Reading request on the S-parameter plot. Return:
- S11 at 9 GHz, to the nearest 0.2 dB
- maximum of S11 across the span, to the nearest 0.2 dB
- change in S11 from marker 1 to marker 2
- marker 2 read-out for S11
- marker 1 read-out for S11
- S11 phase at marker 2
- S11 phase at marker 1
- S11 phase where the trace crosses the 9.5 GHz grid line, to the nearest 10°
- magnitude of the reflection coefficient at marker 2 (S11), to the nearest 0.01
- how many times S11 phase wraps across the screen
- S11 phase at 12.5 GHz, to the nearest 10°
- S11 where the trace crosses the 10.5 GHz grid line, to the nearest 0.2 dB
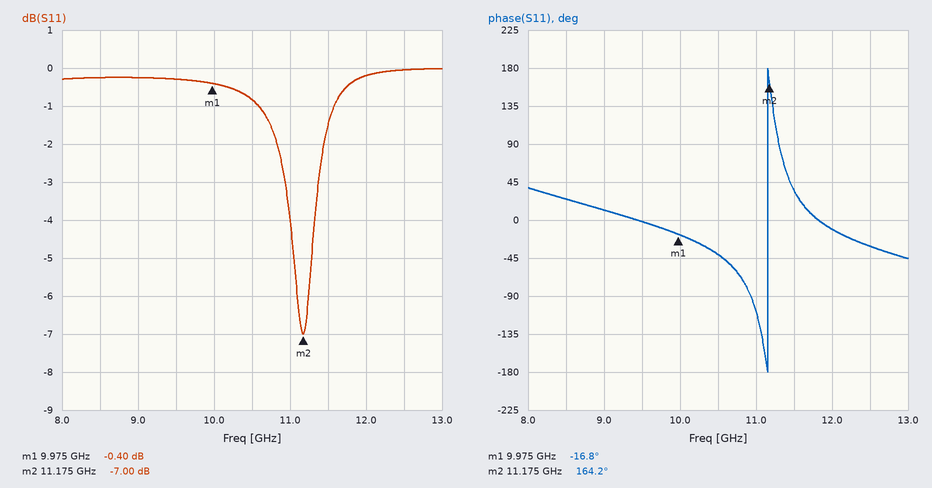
-0.2 dB
0.0 dB
-6.60 dB
-7.00 dB
-0.40 dB
164.2°
-16.8°
0°
0.45
1
-30°
-0.8 dB
